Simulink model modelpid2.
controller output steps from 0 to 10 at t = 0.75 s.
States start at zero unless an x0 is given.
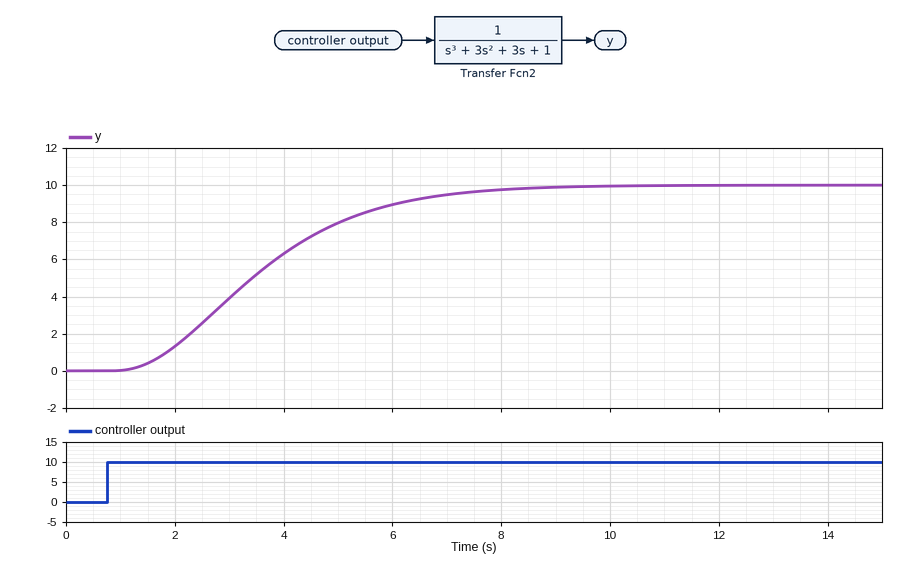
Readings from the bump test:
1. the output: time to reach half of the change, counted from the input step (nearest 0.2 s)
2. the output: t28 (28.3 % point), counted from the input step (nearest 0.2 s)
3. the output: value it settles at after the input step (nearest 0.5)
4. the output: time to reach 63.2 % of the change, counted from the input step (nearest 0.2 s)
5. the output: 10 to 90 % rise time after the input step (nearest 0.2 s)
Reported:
2.6 s
1.8 s
10.0
3.2 s
4.2 s
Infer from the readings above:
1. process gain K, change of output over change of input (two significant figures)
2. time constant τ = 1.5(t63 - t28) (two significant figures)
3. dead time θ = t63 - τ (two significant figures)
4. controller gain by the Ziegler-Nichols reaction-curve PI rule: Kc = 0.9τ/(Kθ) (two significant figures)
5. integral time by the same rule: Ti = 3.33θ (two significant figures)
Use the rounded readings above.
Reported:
1.0
2.1 s
1.1 s
1.7
3.7 s
